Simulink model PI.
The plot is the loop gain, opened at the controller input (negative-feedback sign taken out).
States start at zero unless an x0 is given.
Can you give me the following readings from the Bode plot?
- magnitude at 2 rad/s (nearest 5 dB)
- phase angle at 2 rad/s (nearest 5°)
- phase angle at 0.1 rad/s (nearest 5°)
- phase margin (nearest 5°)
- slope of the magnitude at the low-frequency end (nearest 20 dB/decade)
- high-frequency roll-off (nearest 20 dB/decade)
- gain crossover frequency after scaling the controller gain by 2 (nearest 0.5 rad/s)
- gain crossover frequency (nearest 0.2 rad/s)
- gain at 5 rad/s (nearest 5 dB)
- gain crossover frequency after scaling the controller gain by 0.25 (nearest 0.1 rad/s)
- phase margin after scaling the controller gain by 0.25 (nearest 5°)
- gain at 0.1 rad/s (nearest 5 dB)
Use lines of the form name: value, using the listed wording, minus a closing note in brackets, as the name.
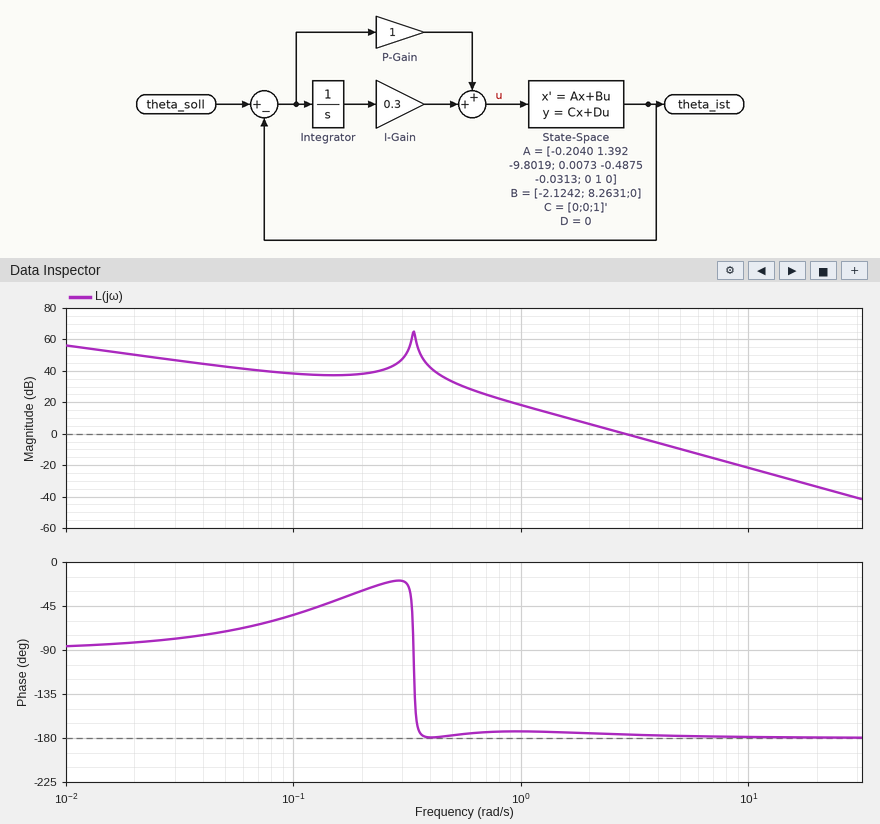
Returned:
magnitude at 2 rad/s: 5 dB
phase angle at 2 rad/s: -175°
phase angle at 0.1 rad/s: -55°
phase margin: 5°
slope of the magnitude at the low-frequency end: -20 dB/decade
high-frequency roll-off: -40 dB/decade
gain crossover frequency after scaling the controller gain by 2: 4.0 rad/s
gain crossover frequency: 2.8 rad/s
gain at 5 rad/s: -10 dB
gain crossover frequency after scaling the controller gain by 0.25: 1.4 rad/s
phase margin after scaling the controller gain by 0.25: 5°
gain at 0.1 rad/s: 40 dB
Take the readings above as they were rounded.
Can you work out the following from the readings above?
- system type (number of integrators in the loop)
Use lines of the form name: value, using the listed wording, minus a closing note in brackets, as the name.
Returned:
system type: 1
